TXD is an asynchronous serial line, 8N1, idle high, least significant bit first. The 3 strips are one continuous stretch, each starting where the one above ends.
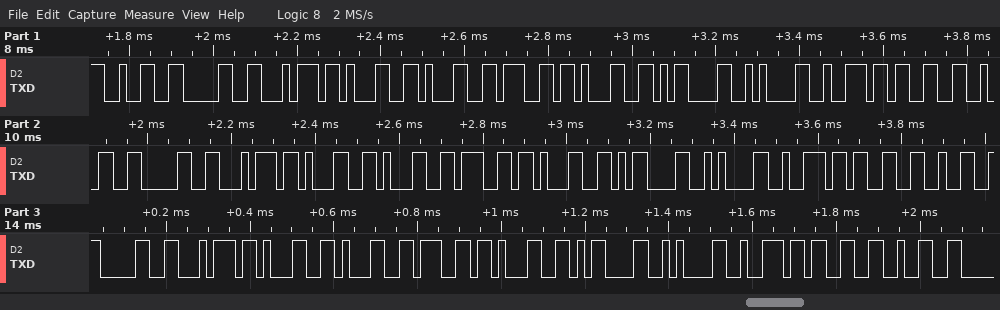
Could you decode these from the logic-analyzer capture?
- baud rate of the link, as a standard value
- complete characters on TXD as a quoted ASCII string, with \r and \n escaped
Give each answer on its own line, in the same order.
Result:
57600 baud
"20t11g1\r\nr320t11g1\r\nr320t11g1\r\nr32"
